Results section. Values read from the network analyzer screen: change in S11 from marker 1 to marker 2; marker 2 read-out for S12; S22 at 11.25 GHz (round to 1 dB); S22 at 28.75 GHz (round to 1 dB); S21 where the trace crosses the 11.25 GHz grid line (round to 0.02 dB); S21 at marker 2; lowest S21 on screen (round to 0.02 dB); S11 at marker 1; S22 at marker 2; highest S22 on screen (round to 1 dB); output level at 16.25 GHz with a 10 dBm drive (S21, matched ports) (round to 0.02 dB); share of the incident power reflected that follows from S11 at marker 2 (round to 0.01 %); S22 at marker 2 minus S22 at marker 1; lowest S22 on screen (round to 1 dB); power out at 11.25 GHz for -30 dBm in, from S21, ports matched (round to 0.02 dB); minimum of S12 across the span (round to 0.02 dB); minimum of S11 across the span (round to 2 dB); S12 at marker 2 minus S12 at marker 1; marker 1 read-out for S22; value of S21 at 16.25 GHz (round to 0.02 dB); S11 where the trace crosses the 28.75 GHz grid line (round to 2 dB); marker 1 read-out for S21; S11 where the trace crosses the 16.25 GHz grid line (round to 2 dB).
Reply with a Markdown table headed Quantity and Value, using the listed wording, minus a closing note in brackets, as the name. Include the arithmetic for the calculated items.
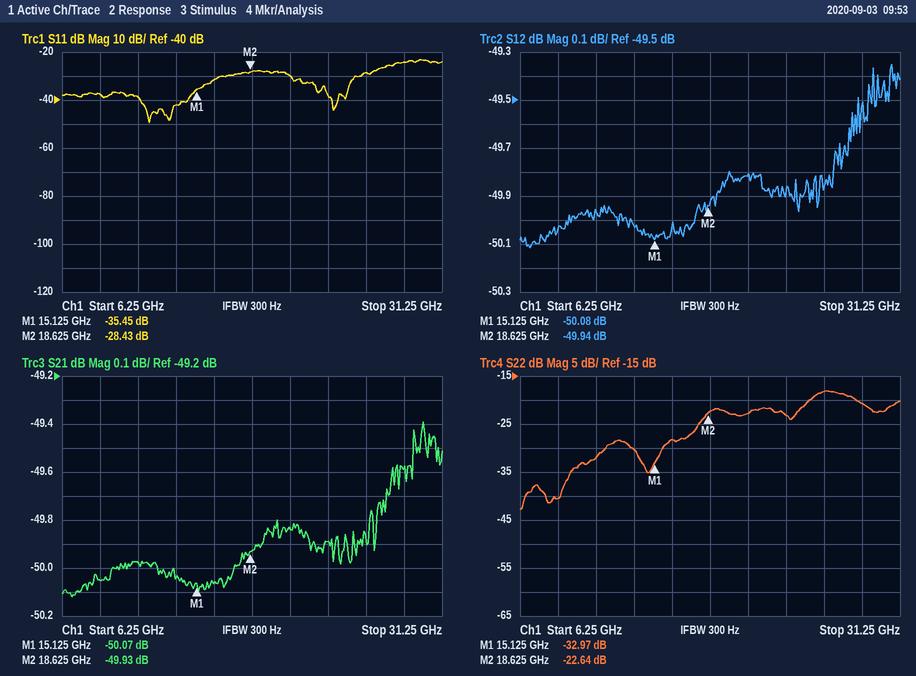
| Quantity | Value |
|---|---|
| change in S11 from marker 1 to marker 2 | -28.43 − (-35.45) = 7.02 dB |
| marker 2 read-out for S12 | -49.94 dB |
| S22 at 11.25 GHz | -32 dB |
| S22 at 28.75 GHz | -21 dB |
| S21 where the trace crosses the 11.25 GHz grid line | -49.98 dB |
| S21 at marker 2 | -49.93 dB |
| lowest S21 on screen | -50.12 dB |
| S11 at marker 1 | -35.45 dB |
| S22 at marker 2 | -22.64 dB |
| highest S22 on screen | -18 dB |
| output level at 16.25 GHz with a 10 dBm drive (S21, matched ports) | 10 dBm + (-50.06 dB) = -40.06 dBm |
| share of the incident power reflected that follows from S11 at marker 2 | 10^(-28.43/10) ≈ 0.14 % |
| S22 at marker 2 minus S22 at marker 1 | -22.64 − (-32.97) = 10.33 dB |
| lowest S22 on screen | -43 dB |
| power out at 11.25 GHz for -30 dBm in, from S21, ports matched | -30 dBm + (-49.98 dB) = -79.98 dBm |
| minimum of S12 across the span | -50.12 dB |
| minimum of S11 across the span | -50 dB |
| S12 at marker 2 minus S12 at marker 1 | -49.94 − (-50.08) = 0.14 dB |
| marker 1 read-out for S22 | -32.97 dB |
| value of S21 at 16.25 GHz | -50.06 dB |
| S11 where the trace crosses the 28.75 GHz grid line | -24 dB |
| marker 1 read-out for S21 | -50.07 dB |
| S11 where the trace crosses the 16.25 GHz grid line | -32 dB |
